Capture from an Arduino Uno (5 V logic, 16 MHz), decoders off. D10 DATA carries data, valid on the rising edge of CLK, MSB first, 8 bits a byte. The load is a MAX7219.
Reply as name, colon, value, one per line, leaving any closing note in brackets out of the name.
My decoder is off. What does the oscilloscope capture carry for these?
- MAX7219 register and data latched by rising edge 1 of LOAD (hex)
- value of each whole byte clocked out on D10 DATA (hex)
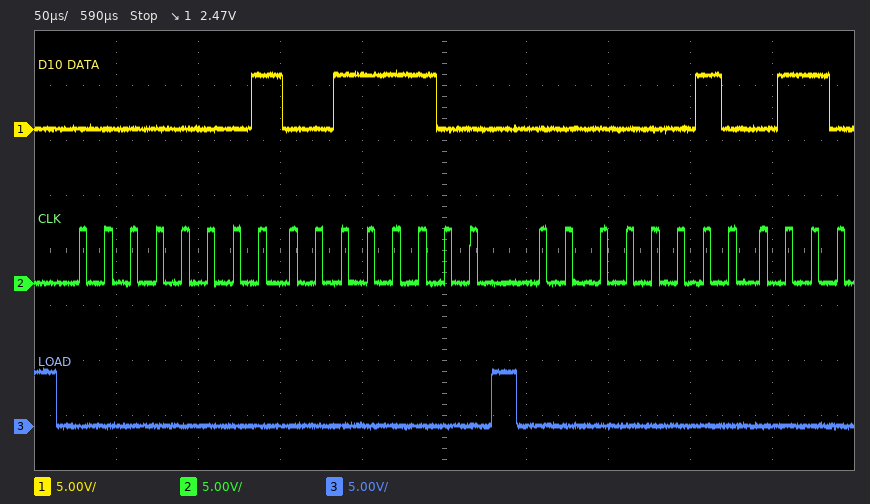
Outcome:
MAX7219 register and data latched by rising edge 1 of LOAD: register 0x1, data 0x3C
value of each whole byte clocked out on D10 DATA: 01 3C 02
